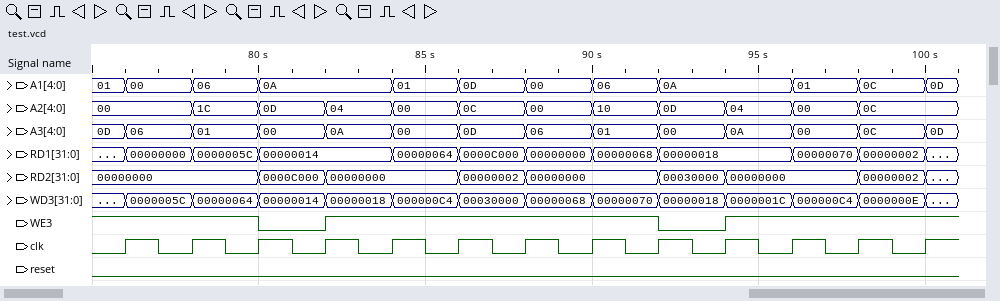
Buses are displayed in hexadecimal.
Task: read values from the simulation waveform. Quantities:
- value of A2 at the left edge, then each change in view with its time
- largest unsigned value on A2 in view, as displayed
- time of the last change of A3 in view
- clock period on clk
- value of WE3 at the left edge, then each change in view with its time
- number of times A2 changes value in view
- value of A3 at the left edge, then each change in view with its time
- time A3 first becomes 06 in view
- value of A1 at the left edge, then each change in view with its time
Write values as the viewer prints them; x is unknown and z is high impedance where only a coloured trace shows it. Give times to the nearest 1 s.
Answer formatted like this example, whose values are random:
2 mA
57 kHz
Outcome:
00, 1C at 78 s, 0D at 80 s, 04 at 82 s, 00 at 84 s, 0C at 86 s, 00 at 88 s, 10 at 90 s, 0D at 92 s, 04 at 94 s, 00 at 96 s, 0C at 98 s
1C
100 s
2 s
1, 0 at 80 s, 1 at 82 s, 0 at 92 s, 1 at 94 s
11
0D, 06 at 76 s, 01 at 78 s, 00 at 80 s, 0A at 82 s, 00 at 84 s, 0D at 86 s, 06 at 88 s, 01 at 90 s, 00 at 92 s, 0A at 94 s, 00 at 96 s, 0C at 98 s, 0D at 100 s
76 s
01, 00 at 76 s, 06 at 78 s, 0A at 80 s, 01 at 84 s, 0D at 86 s, 00 at 88 s, 06 at 90 s, 0A at 92 s, 01 at 96 s, 0C at 98 s, 0D at 100 s
